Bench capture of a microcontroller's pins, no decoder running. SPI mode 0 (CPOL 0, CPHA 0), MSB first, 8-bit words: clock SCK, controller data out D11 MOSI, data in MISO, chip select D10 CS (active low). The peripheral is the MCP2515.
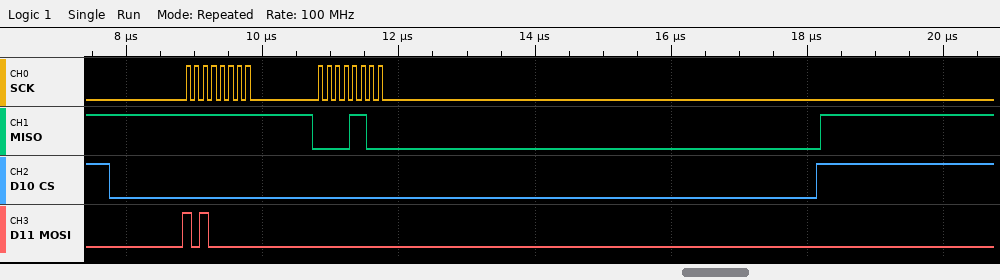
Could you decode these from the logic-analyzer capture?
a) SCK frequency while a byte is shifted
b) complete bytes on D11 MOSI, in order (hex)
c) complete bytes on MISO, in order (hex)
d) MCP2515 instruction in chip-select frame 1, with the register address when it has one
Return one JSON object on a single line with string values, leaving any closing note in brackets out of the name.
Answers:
{"SCK frequency while a byte is shifted": "8 MHz", "complete bytes on D11 MOSI, in order": "A0 00", "complete bytes on MISO, in order": "FF 0C", "MCP2515 instruction in chip-select frame 1, with the register address when it has one": "READ STATUS"}
